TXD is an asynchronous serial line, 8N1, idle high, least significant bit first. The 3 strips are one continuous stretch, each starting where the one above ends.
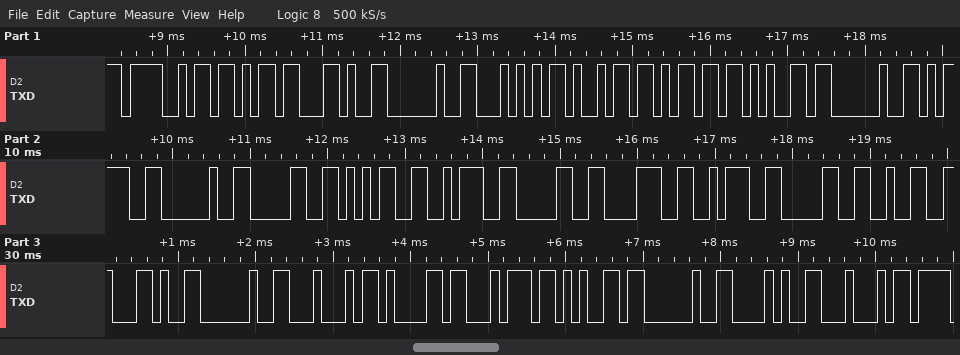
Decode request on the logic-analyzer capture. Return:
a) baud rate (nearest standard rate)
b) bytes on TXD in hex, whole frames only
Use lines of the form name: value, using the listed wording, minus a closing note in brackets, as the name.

baud rate: 9600 baud
bytes on TXD in hex, whole frames only: 4F 6B 2C 20 54 69 6D 65 20 3D 20 30 35 3A 30 38 3A 30 32 2C 20 44 61 74 65 20 28 44
